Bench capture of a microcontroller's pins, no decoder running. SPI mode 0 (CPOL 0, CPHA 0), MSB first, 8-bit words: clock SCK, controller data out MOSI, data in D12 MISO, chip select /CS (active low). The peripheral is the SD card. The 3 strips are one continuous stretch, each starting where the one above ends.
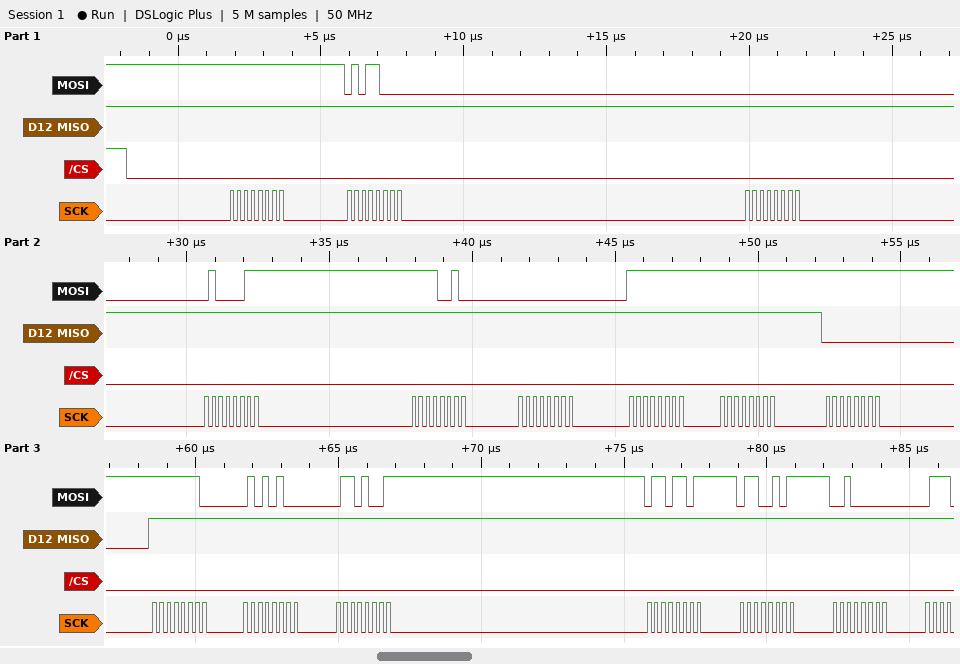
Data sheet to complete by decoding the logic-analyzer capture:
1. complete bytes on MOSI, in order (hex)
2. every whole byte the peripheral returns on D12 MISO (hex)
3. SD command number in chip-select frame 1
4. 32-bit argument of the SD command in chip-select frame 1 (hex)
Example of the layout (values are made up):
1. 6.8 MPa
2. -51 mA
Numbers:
1. FF 58 00 43 F2 00 FF FF FF FE 54 69 6D 65 20
2. FF FF FF FF FF FF FF FF 00 FF FF FF FF FF FF
3. CMD24
4. 0x0043F200
